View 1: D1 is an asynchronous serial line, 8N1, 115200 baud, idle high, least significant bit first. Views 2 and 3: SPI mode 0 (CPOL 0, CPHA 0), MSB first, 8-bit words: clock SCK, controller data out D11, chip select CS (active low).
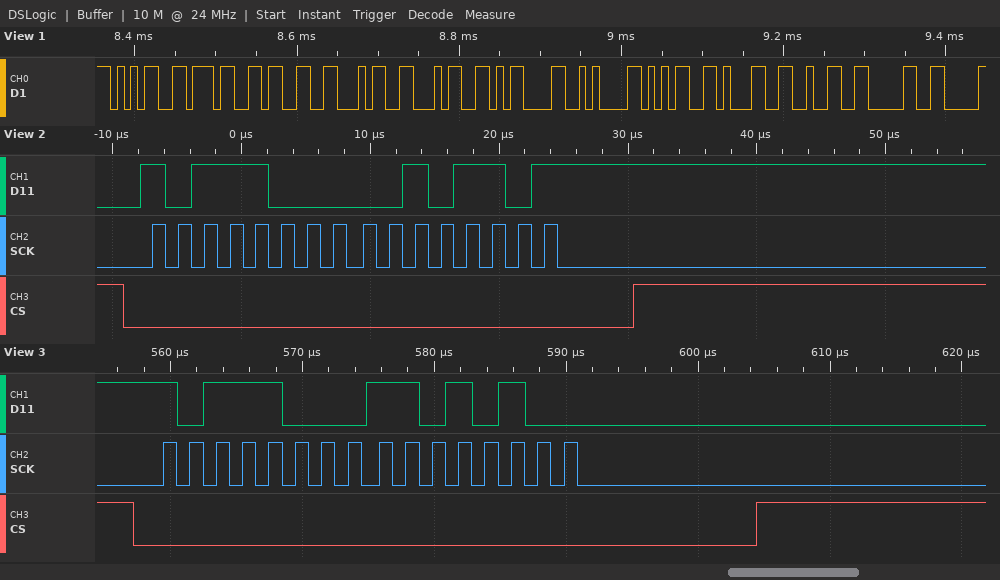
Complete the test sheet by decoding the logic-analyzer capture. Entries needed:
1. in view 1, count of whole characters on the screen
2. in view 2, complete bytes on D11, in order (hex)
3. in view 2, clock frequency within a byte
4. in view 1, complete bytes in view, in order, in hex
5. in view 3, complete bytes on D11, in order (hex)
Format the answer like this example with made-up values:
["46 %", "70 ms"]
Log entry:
["11", "0xB8 0x2D", "500 kHz", "35 37 33 34 34 0D 0A 35 31 32 30", "B8 D4"]
